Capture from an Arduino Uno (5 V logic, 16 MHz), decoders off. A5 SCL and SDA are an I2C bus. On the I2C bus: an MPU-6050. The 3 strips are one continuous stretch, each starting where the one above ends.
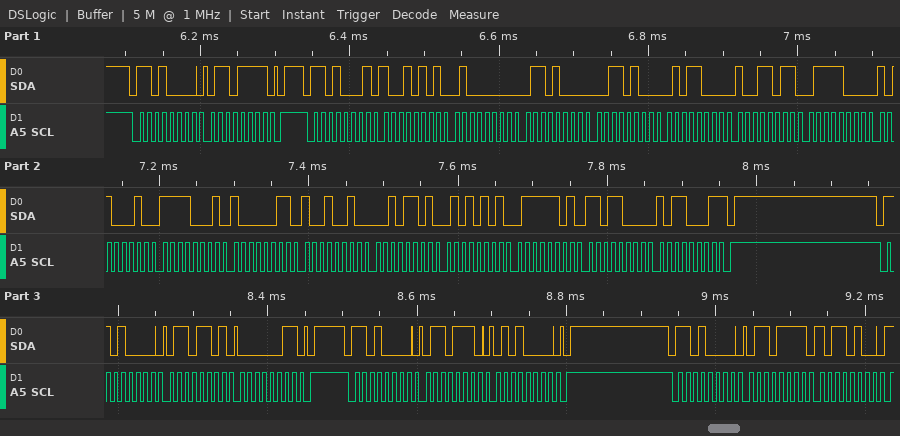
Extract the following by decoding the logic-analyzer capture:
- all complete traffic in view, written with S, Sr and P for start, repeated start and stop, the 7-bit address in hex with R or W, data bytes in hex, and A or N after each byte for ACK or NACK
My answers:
S 68W A 6F A P S 68R A 95 A 40 A 68 A 34 A 58 A 9B A 78 A A2 A F1 A 83 A 92 A 2D A 55 A 7D A D8 A B1 N P S 68W A 6D A 03 A P S 68W A 6E A 50 A P S 68W A 6F A B4 A
